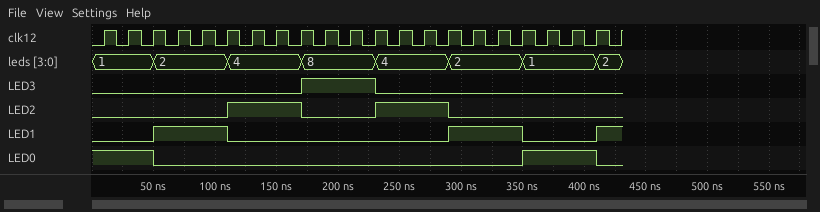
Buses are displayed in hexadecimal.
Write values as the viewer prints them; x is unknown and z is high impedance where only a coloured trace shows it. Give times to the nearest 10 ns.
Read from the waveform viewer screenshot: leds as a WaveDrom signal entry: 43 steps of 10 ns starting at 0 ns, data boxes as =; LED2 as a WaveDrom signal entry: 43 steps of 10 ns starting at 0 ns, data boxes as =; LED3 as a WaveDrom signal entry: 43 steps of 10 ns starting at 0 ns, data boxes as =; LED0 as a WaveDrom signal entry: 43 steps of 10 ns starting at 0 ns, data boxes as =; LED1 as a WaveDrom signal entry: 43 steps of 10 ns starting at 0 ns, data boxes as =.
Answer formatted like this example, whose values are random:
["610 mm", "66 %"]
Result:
["{name: 'leds', wave: '=....=.....=.....=.....=.....=.....=.....=.', data: '1 2 4 8 4 2 1 2'}", "{name: 'LED2', wave: '0..........1.....0.....1.....0.............'}", "{name: 'LED3', wave: '0................1.....0...................'}", "{name: 'LED0', wave: '1....0.............................1.....0.'}", "{name: 'LED1', wave: '0....1.....0.................1.....0.....1.'}"]
